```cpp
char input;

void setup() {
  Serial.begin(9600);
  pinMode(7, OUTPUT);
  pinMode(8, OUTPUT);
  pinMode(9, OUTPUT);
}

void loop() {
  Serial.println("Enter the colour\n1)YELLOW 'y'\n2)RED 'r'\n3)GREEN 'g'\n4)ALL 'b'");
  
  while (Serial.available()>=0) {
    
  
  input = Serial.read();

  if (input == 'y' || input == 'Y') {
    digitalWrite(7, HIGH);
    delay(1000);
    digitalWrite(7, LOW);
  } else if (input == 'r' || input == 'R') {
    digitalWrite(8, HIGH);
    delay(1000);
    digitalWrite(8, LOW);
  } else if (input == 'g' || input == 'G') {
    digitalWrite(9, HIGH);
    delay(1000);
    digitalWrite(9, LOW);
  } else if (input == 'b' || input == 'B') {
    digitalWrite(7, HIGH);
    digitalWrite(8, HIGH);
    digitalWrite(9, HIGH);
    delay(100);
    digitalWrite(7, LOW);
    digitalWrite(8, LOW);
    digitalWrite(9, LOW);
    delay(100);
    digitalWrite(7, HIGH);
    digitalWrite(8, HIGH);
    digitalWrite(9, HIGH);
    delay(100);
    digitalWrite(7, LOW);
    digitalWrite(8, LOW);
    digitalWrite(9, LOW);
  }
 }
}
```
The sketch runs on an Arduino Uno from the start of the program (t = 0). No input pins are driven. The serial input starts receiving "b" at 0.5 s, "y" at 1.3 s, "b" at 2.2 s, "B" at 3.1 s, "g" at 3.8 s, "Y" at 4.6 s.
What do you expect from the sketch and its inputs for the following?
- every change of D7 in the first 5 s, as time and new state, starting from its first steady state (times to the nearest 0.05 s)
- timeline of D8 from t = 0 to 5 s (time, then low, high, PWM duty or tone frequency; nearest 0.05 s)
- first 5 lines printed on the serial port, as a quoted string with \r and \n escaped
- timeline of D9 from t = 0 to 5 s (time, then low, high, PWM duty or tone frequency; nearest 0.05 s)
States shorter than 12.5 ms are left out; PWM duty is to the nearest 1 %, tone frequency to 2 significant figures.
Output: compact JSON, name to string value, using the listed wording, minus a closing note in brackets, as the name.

{"every change of D7 in the first 5 s, as time and new state, starting from its first steady state": "0 s low; 0.5 s high; 0.6 s low; 0.7 s high; 0.8 s low; 1.3 s high; 2.4 s low; 2.5 s high; 2.6 s low; 3.1 s high; 3.2 s low; 3.3 s high; 3.4 s low; 4.8 s high", "timeline of D8 from t = 0 to 5 s": "0 s low; 0.5 s high; 0.6 s low; 0.7 s high; 0.8 s low; 2.3 s high; 2.4 s low; 2.5 s high; 2.6 s low; 3.1 s high; 3.2 s low; 3.3 s high; 3.4 s low", "first 5 lines printed on the serial port, as a quoted string with \\r and \\n escaped": "\"Enter the colour\\n1)YELLOW 'y'\\n2)RED 'r'\\n3)GREEN 'g'\\n4)ALL 'b'\\r\\n\"", "timeline of D9 from t = 0 to 5 s": "0 s low; 0.5 s high; 0.6 s low; 0.7 s high; 0.8 s low; 2.3 s high; 2.4 s low; 2.5 s high; 2.6 s low; 3.1 s high; 3.2 s low; 3.3 s high; 3.4 s low; 3.8 s high; 4.8 s low"}
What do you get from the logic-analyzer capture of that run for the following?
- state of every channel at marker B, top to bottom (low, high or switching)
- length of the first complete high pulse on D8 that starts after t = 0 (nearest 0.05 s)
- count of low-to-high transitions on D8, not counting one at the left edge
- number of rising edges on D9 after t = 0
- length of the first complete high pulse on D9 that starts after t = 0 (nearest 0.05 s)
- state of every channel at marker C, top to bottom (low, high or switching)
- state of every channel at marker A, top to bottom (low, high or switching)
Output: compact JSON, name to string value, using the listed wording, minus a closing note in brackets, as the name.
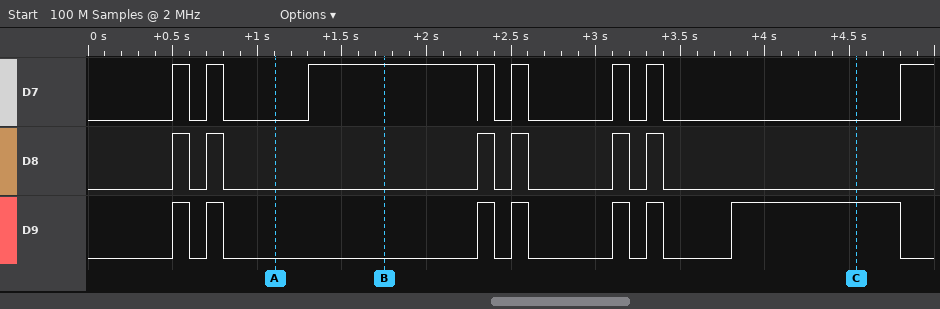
{"state of every channel at marker B, top to bottom": "D7 high, D8 low, D9 low", "length of the first complete high pulse on D8 that starts after t = 0": "0.10 s", "count of low-to-high transitions on D8, not counting one at the left edge": "6", "number of rising edges on D9 after t = 0": "7", "length of the first complete high pulse on D9 that starts after t = 0": "0.10 s", "state of every channel at marker C, top to bottom": "D7 low, D8 low, D9 high", "state of every channel at marker A, top to bottom": "D7 low, D8 low, D9 low"}
